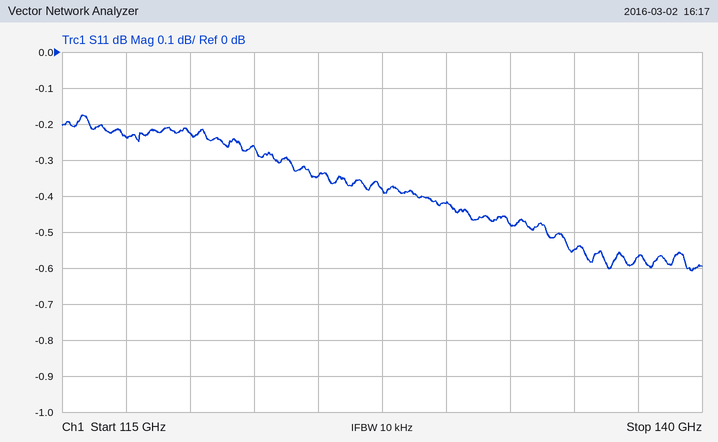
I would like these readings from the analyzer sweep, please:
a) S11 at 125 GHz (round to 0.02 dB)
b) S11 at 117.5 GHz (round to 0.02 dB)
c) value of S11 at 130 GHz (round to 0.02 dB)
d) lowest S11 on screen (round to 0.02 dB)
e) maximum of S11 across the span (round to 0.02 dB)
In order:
-0.34 dB
-0.24 dB
-0.42 dB
-0.60 dB
-0.18 dB
